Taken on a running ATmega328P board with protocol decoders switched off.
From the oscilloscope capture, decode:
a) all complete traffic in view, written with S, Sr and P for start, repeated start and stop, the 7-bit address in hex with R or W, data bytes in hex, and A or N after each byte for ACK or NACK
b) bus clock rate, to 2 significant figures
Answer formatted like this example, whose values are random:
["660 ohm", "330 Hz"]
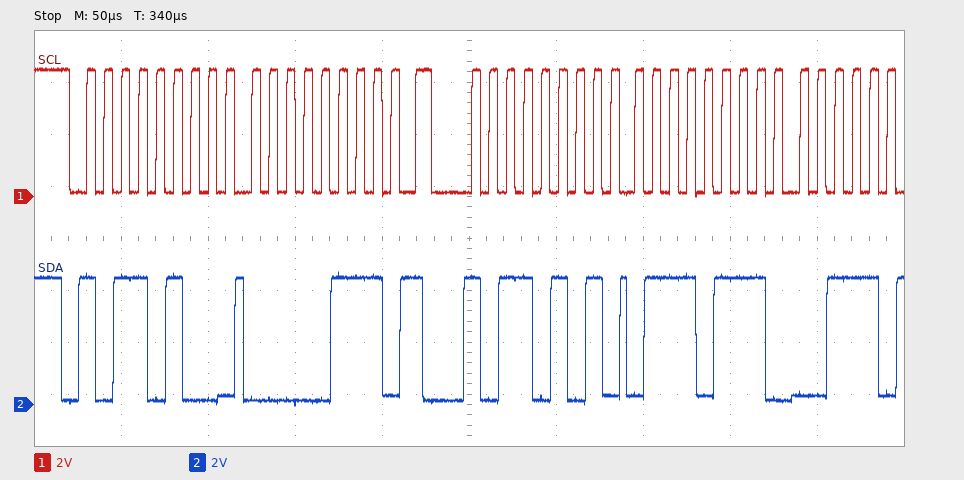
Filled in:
["S 5AW A 07 A Sr 5AR A 77 A", "100 kHz"]
